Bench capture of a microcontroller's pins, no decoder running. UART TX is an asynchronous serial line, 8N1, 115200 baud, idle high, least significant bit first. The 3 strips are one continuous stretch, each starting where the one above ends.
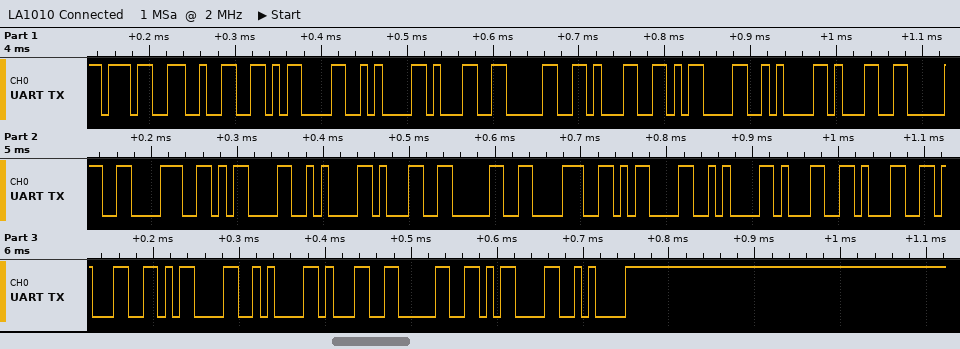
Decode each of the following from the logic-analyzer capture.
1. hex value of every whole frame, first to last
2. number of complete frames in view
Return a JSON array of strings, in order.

["37 32 0D 0A 31 30 31 0D 0A 31 30 38 0D 0A 31 30 38 0D 0A 31 31 31 0D 0A 31 30 0D 0A", "28"]
